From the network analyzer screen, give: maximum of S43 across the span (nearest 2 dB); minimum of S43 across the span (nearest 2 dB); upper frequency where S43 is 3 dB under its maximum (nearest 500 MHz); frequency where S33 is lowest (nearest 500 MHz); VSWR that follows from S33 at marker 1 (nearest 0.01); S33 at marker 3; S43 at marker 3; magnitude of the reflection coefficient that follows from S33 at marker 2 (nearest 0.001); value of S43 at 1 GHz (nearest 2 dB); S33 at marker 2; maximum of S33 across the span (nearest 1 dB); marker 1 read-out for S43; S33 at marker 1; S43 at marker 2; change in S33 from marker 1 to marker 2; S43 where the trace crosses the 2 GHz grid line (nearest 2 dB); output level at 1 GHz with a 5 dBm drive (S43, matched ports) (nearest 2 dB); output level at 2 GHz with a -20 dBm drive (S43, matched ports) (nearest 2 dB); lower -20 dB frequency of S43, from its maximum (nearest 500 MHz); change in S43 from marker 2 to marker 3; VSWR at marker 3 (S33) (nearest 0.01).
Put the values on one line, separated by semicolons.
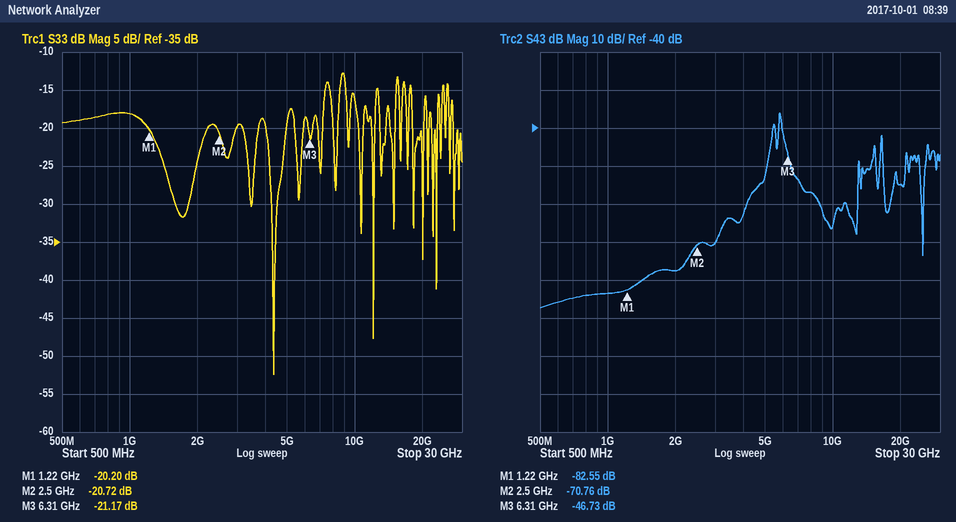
-36 dB; -88 dB; 6.0 GHz; 4.5 GHz; 1.22; -21.17 dB; -46.73 dB; 0.092; -84 dB; -20.72 dB; -13 dB; -82.55 dB; -20.20 dB; -70.76 dB; -0.52 dB; -78 dB; -78 dBm; -98 dBm; 4.5 GHz; 24.03 dB; 1.19
